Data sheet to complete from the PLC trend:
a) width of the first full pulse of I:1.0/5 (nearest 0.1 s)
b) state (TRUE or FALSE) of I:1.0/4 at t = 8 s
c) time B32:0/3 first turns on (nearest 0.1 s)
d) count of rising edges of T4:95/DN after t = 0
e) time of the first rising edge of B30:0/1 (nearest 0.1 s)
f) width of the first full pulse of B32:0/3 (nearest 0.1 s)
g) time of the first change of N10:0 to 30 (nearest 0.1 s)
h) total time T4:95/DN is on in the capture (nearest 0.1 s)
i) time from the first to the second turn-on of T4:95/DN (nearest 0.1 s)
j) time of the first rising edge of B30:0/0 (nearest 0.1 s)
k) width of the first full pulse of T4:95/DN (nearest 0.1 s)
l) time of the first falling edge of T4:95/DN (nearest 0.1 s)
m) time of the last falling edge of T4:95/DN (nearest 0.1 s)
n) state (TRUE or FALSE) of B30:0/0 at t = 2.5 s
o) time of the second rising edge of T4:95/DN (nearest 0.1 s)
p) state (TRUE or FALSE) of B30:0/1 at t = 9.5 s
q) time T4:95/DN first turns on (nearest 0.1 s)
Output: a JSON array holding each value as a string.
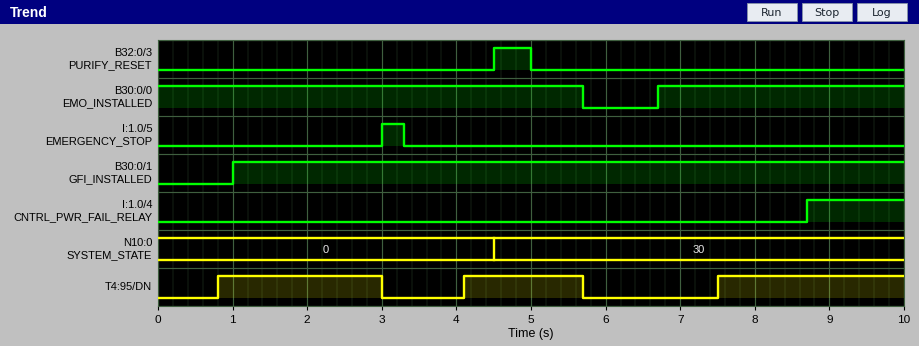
["0.3 s", "FALSE", "4.5 s", "3", "1.0 s", "0.5 s", "4.5 s", "6.3 s", "3.3 s", "6.7 s", "2.2 s", "3.0 s", "5.7 s", "TRUE", "4.1 s", "TRUE", "0.8 s"]
